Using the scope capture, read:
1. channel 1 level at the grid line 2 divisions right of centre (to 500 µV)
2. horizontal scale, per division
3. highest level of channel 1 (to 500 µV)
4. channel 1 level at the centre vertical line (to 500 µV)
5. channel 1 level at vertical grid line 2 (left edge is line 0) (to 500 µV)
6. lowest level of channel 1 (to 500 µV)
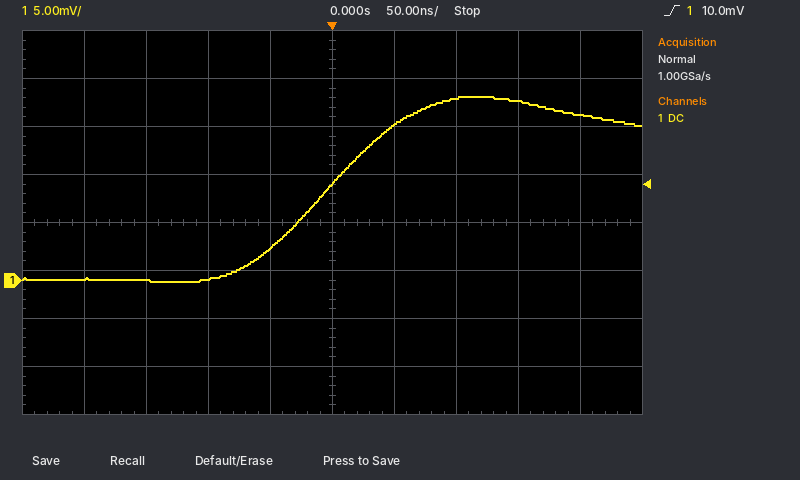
19.0 mV
50 ns
19.0 mV
10.0 mV
0.0 mV
0.0 mV
